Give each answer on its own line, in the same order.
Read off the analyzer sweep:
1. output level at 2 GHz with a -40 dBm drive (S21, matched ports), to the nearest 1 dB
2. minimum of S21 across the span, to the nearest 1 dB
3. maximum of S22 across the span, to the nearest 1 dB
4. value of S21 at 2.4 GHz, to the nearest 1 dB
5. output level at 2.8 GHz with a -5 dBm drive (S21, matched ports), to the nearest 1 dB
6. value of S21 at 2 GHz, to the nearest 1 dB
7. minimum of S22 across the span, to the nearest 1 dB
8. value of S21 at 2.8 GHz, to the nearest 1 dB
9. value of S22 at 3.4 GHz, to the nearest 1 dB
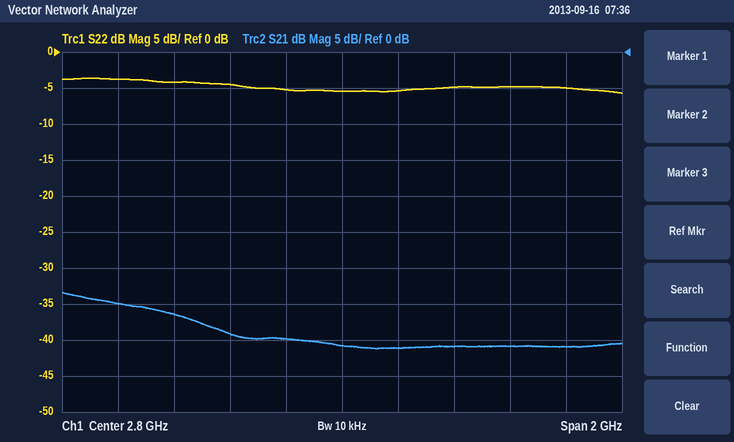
-75 dBm
-41 dB
-4 dB
-39 dB
-46 dBm
-35 dB
-6 dB
-41 dB
-5 dB
